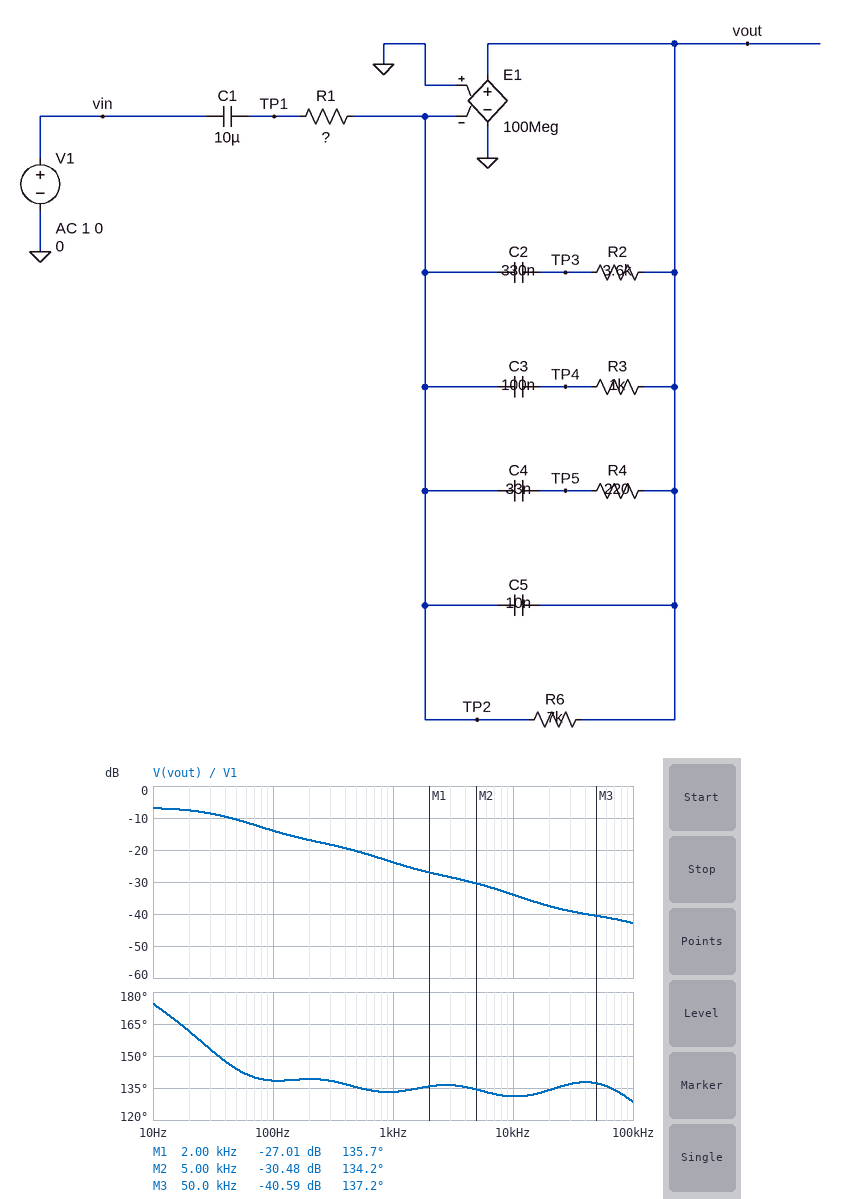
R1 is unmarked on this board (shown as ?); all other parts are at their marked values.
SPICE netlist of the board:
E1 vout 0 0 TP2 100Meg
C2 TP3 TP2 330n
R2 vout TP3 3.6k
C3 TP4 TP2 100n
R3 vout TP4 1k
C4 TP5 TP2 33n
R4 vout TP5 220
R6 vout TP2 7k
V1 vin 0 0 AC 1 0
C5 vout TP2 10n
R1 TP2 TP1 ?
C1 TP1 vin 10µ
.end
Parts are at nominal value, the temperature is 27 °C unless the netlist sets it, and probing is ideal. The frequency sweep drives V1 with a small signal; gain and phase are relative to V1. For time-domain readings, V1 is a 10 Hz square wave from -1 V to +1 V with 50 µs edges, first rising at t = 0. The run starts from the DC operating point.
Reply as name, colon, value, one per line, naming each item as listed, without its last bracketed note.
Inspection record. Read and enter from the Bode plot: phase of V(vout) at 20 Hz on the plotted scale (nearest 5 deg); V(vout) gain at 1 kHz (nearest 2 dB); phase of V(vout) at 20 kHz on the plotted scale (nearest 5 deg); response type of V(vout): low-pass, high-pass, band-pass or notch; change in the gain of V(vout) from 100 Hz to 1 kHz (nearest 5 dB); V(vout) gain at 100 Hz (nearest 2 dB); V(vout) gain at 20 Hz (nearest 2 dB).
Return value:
phase of V(vout) at 20 Hz on the plotted scale: 160 deg
V(vout) gain at 1 kHz: -24 dB
phase of V(vout) at 20 kHz on the plotted scale: 135 deg
response type of V(vout): low-pass, high-pass, band-pass or notch: low-pass
change in the gain of V(vout) from 100 Hz to 1 kHz: -10 dB
V(vout) gain at 100 Hz: -14 dB
V(vout) gain at 20 Hz: -8 dB
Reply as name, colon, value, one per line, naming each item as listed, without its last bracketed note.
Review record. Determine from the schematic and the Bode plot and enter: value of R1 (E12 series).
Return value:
value of R1: 15 kΩ
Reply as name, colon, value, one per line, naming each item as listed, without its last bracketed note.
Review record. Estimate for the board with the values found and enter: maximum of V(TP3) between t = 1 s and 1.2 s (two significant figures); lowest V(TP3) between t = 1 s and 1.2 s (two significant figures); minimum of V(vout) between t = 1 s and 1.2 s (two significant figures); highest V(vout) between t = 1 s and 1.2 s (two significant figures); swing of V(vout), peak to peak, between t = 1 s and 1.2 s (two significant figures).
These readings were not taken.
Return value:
maximum of V(TP3) between t = 1 s and 1.2 s: 480 mV
lowest V(TP3) between t = 1 s and 1.2 s: -480 mV
minimum of V(vout) between t = 1 s and 1.2 s: -480 mV
highest V(vout) between t = 1 s and 1.2 s: 480 mV
swing of V(vout), peak to peak, between t = 1 s and 1.2 s: 970 mV
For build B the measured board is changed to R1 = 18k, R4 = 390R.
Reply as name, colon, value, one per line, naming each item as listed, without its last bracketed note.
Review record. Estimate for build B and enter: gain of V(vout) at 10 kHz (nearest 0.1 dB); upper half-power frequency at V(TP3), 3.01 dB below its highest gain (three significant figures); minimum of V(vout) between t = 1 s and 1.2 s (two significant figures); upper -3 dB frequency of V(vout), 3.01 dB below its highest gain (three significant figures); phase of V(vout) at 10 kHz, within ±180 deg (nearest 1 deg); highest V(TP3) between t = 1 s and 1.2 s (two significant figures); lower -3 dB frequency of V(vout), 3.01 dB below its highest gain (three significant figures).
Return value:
gain of V(vout) at 10 kHz: -35.1 dB
upper half-power frequency at V(TP3), 3.01 dB below its highest gain: 39.1 Hz
minimum of V(vout) between t = 1 s and 1.2 s: -400 mV
upper -3 dB frequency of V(vout), 3.01 dB below its highest gain: 42.6 Hz
phase of V(vout) at 10 kHz, within ±180 deg: 140 deg
highest V(TP3) between t = 1 s and 1.2 s: 400 mV
lower -3 dB frequency of V(vout), 3.01 dB below its highest gain: 847 mHz
